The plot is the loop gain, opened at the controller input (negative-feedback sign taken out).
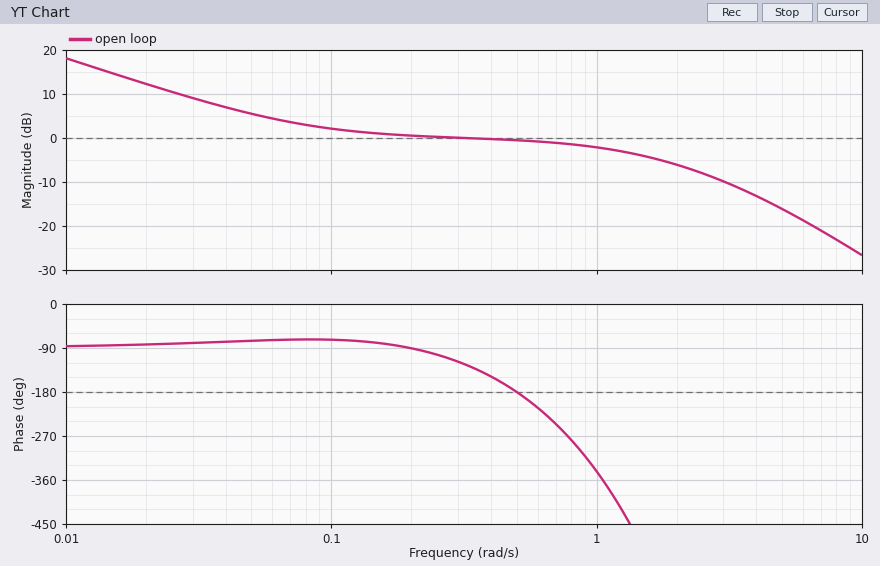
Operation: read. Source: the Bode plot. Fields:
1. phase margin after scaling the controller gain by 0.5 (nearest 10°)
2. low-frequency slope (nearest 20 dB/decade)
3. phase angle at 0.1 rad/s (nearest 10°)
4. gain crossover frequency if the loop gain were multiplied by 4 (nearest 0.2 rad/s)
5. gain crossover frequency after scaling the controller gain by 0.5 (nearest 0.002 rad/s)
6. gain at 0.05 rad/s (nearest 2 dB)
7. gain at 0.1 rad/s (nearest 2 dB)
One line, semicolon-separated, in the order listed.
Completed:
100°; -20 dB/decade; -70°; 3.6 rad/s; 0.046 rad/s; 6 dB; 2 dB
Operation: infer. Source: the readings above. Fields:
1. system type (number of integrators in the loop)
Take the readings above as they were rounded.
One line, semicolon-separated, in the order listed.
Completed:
1
